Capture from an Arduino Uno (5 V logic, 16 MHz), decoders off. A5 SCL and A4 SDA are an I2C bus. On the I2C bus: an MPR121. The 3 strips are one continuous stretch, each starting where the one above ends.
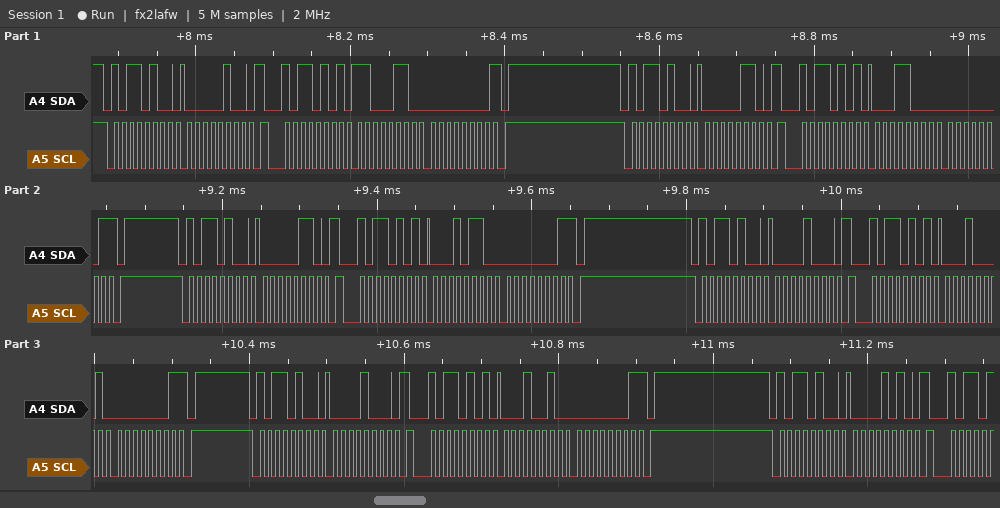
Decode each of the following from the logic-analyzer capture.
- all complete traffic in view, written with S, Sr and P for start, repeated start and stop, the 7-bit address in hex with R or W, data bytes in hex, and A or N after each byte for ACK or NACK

S 5AW A 04 A Sr 5AR A C6 A 00 N P S 5AW A 06 A Sr 5AR A 18 A 01 N P S 5AW A 06 A Sr 5AR A 16 A 01 N P S 5AW A 08 A Sr 5AR A 11 A 01 N P S 5AW A 08 A Sr 5AR A 12 A 01 N P S 5AW A 0A A
